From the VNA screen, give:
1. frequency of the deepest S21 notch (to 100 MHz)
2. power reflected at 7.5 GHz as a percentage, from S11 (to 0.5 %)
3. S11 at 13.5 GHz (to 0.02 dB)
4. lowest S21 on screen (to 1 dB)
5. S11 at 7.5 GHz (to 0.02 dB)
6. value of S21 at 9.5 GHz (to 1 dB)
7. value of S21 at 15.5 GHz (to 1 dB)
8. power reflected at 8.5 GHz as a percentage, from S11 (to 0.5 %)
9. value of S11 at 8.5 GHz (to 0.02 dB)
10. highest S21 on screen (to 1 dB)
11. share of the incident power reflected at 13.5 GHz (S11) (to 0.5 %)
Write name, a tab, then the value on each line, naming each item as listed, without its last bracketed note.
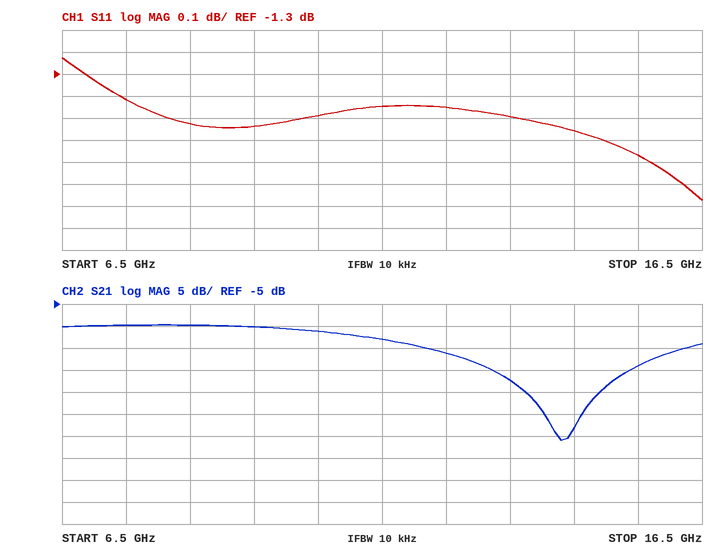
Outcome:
frequency of the deepest S21 notch	14.3 GHz
power reflected at 7.5 GHz as a percentage, from S11	72.0 %
S11 at 13.5 GHz	-1.50 dB
lowest S21 on screen	-36 dB
S11 at 7.5 GHz	-1.42 dB
value of S21 at 9.5 GHz	-10 dB
value of S21 at 15.5 GHz	-19 dB
power reflected at 8.5 GHz as a percentage, from S11	70.5 %
value of S11 at 8.5 GHz	-1.52 dB
highest S21 on screen	-10 dB
share of the incident power reflected at 13.5 GHz (S11)	71.0 %
